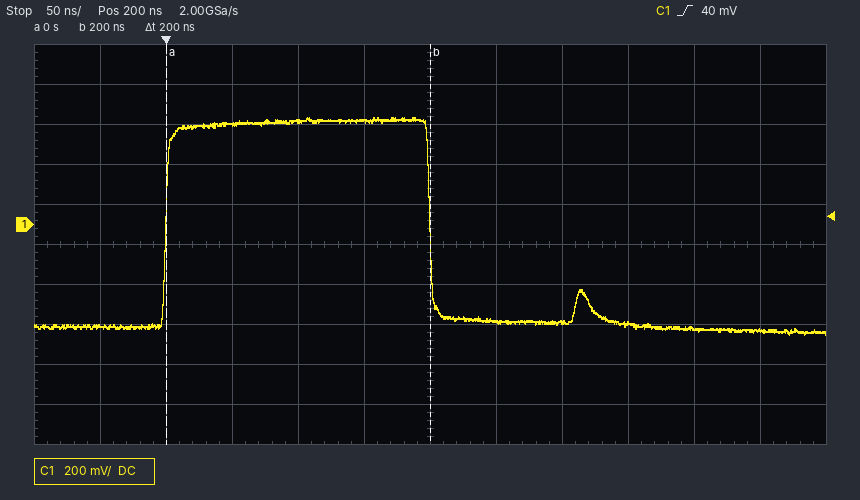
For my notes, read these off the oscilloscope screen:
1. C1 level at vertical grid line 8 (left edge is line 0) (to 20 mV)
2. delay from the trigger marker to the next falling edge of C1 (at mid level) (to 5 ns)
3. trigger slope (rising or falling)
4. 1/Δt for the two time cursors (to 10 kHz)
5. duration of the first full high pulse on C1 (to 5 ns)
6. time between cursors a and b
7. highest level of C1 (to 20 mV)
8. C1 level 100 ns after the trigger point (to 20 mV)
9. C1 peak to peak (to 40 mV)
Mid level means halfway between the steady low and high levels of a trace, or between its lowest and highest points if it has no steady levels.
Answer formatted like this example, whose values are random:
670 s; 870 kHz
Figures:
-480 mV; 200 ns; rising; 5.00 MHz; 200 ns; 200 ns; 540 mV; 520 mV; 1.08 V
